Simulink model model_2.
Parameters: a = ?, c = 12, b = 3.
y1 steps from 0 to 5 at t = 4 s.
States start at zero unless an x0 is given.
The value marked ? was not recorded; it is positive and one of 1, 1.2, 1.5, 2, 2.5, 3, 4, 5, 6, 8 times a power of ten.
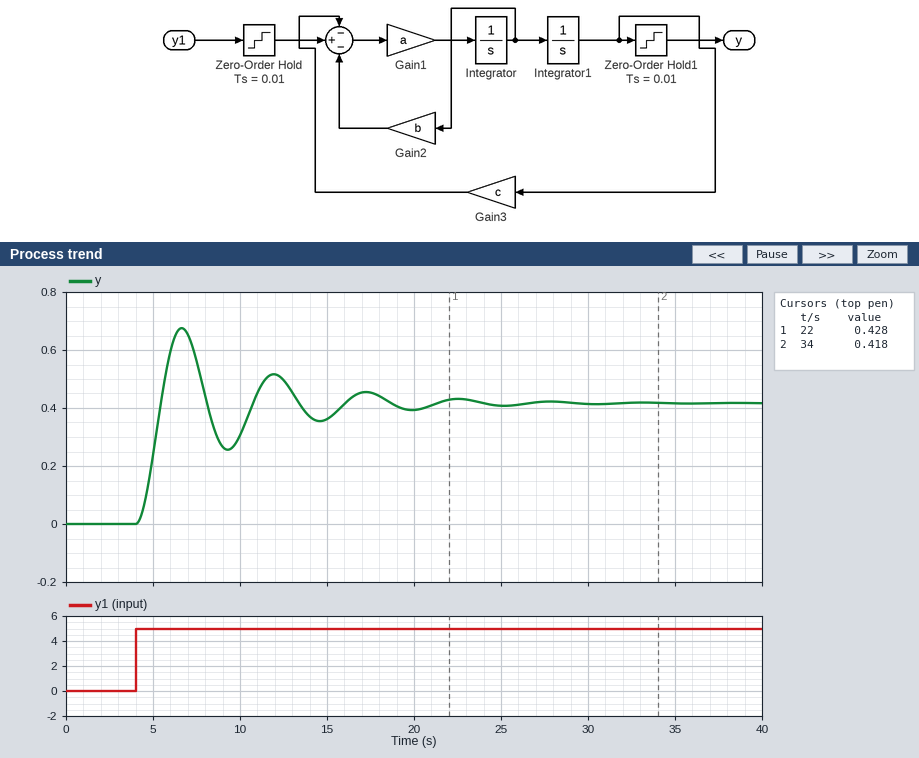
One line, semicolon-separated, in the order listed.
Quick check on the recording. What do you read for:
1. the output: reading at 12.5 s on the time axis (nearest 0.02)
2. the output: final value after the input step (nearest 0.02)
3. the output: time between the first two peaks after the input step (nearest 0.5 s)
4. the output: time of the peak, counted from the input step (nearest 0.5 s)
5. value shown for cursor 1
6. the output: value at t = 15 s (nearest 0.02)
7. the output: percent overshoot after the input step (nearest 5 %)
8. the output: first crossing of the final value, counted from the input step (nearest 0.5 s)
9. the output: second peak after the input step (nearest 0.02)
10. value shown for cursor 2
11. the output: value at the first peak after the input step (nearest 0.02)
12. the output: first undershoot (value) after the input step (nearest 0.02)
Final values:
0.50; 0.42; 5.5 s; 2.5 s; 0.428; 0.36; 60 %; 1.5 s; 0.52; 0.418; 0.68; 0.26
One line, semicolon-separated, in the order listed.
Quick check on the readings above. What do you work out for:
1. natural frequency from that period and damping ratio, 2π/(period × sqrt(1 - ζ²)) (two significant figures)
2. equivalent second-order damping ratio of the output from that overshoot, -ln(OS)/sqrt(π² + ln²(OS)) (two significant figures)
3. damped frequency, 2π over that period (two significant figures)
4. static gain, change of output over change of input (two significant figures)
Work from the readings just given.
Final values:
1.2 rad/s; 0.16; 1.1 rad/s; 0.084
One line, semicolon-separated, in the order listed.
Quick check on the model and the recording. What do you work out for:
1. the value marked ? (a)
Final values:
0.12
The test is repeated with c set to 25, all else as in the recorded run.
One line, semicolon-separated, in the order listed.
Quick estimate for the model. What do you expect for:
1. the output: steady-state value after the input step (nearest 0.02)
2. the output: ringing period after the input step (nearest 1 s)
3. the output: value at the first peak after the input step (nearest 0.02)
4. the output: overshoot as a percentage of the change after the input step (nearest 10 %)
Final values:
0.20; 4 s; 0.34; 70 %
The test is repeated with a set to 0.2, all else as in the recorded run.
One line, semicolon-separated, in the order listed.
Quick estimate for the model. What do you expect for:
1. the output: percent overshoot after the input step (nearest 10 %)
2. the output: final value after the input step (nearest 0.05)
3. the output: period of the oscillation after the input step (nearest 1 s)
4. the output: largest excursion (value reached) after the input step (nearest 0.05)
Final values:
50 %; 0.40; 4 s; 0.65
